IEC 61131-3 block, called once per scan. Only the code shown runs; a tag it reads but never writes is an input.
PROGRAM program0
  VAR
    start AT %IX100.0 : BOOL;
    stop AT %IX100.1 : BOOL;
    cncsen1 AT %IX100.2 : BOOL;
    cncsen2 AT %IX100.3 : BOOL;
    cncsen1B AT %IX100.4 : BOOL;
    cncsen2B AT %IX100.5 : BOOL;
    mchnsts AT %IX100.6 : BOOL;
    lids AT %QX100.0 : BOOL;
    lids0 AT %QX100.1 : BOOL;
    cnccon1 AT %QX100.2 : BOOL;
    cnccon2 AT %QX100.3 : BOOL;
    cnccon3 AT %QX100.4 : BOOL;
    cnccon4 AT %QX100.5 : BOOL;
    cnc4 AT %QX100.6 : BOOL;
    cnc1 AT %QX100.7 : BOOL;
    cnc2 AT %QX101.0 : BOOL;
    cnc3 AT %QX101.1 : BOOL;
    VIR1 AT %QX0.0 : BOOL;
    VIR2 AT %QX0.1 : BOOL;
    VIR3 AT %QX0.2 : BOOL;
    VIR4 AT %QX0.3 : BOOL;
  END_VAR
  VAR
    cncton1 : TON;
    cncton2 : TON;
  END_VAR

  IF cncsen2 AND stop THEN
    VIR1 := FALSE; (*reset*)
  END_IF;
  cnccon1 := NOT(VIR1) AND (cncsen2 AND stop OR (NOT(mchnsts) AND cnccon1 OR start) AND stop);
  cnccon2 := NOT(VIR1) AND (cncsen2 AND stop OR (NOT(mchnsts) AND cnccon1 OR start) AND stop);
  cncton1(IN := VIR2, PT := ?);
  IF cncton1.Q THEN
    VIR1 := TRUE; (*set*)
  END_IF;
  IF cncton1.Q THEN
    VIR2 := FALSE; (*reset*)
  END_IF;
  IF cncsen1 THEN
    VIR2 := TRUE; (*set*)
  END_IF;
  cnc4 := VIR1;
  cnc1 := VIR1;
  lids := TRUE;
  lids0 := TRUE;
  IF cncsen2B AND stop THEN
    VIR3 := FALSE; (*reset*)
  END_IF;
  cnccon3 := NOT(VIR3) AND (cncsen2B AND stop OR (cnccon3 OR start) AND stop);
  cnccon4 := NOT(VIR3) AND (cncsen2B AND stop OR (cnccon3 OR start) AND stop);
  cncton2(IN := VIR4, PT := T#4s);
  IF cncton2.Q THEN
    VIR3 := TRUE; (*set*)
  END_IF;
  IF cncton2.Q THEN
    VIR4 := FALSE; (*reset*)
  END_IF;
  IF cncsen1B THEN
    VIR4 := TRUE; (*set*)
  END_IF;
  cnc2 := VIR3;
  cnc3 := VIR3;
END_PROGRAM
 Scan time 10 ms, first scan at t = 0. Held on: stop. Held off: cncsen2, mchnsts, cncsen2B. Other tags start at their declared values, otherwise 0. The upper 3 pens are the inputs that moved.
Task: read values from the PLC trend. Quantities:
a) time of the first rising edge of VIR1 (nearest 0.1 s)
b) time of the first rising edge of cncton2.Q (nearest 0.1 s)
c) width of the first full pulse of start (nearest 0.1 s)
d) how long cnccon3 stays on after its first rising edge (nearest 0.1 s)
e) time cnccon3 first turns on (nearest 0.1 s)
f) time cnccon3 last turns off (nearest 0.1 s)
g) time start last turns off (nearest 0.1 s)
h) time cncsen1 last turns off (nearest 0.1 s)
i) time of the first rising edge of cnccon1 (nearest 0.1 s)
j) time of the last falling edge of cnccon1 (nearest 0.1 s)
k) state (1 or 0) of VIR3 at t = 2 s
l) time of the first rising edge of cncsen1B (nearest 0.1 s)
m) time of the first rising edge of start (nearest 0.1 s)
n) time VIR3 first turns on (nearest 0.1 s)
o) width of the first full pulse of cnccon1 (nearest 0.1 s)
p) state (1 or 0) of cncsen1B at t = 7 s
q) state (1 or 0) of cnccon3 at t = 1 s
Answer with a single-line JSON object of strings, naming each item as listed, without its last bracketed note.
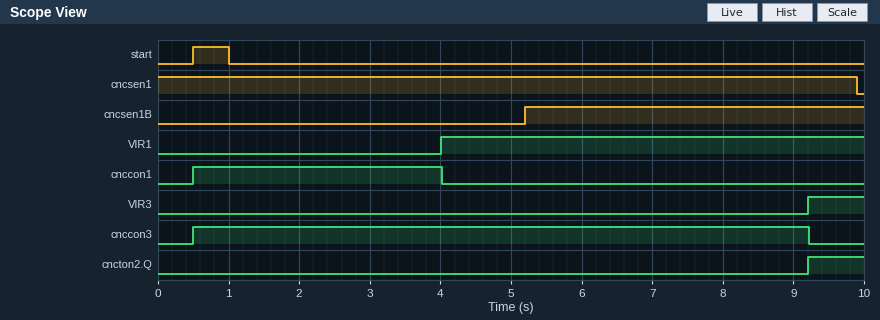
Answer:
{"time of the first rising edge of VIR1": "4.0 s", "time of the first rising edge of cncton2.Q": "9.2 s", "width of the first full pulse of start": "0.5 s", "how long cnccon3 stays on after its first rising edge": "8.7 s", "time cnccon3 first turns on": "0.5 s", "time cnccon3 last turns off": "9.2 s", "time start last turns off": "1.0 s", "time cncsen1 last turns off": "9.9 s", "time of the first rising edge of cnccon1": "0.5 s", "time of the last falling edge of cnccon1": "4.0 s", "state (1 or 0) of VIR3 at t = 2 s": "0", "time of the first rising edge of cncsen1B": "5.2 s", "time of the first rising edge of start": "0.5 s", "time VIR3 first turns on": "9.2 s", "width of the first full pulse of cnccon1": "3.5 s", "state (1 or 0) of cncsen1B at t = 7 s": "1", "state (1 or 0) of cnccon3 at t = 1 s": "1"}
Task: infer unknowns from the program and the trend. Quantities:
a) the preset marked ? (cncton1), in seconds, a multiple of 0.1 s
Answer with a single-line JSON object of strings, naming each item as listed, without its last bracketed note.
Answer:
{"the preset marked ? (cncton1), in seconds, a multiple of 0.1 s": "4.0 s"}
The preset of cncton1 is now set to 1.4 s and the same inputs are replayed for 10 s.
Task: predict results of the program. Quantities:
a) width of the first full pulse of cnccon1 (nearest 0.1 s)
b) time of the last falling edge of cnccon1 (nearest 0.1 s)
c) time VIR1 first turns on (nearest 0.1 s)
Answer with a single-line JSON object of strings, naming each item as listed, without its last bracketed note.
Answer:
{"width of the first full pulse of cnccon1": "0.9 s", "time of the last falling edge of cnccon1": "1.4 s", "time VIR1 first turns on": "1.4 s"}
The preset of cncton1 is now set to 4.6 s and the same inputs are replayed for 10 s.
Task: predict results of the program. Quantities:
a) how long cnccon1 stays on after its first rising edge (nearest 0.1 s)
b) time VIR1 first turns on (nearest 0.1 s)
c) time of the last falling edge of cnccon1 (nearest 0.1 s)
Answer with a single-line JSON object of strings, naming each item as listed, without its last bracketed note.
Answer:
{"how long cnccon1 stays on after its first rising edge": "4.1 s", "time VIR1 first turns on": "4.6 s", "time of the last falling edge of cnccon1": "4.6 s"}
